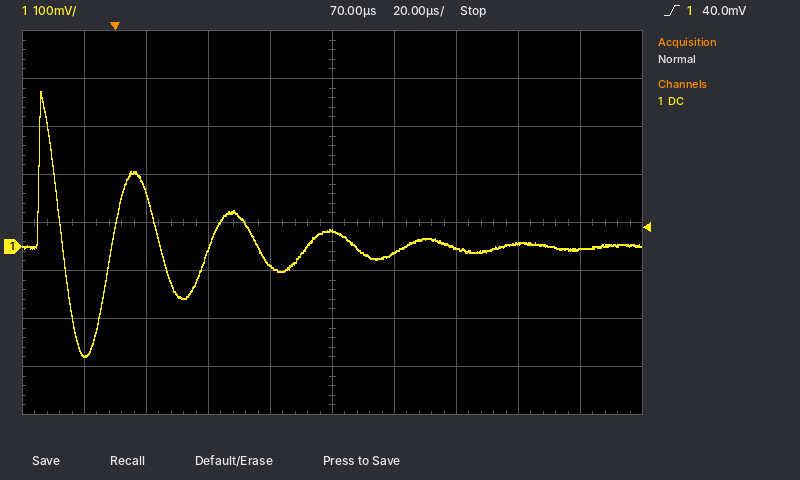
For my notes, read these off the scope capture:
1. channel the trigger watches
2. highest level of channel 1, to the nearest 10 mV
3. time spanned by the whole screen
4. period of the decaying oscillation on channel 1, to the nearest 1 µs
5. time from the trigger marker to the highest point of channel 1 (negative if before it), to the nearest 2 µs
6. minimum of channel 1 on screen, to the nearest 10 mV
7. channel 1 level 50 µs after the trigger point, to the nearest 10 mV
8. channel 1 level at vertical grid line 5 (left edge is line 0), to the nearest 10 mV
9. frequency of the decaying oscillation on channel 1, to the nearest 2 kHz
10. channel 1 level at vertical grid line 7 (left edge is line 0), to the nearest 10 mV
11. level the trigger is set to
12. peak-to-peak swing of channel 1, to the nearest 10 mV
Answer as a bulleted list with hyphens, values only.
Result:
- channel 1
- 320 mV
- 200 µs
- 31 µs
- -24 µs
- -230 mV
- -40 mV
- 30 mV
- 32 kHz
- 0 mV
- 40.0 mV
- 550 mV
